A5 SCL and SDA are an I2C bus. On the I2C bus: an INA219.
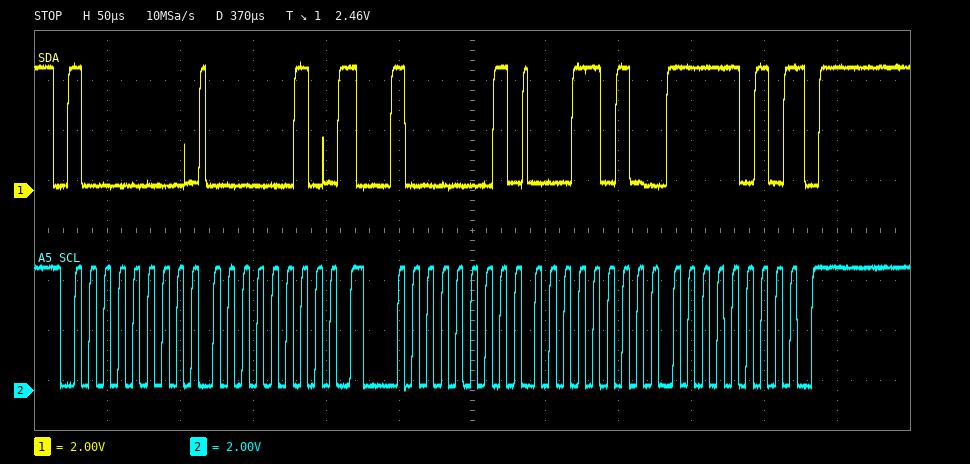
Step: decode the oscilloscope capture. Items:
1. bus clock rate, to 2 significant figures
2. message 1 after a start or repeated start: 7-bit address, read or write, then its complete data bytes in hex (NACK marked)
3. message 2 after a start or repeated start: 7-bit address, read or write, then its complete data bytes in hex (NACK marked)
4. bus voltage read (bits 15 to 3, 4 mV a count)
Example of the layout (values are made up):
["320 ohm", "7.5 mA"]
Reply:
["100 kHz", "0x40 write: 02", "0x40 read: 1A FA NACK", "3.452 V"]
